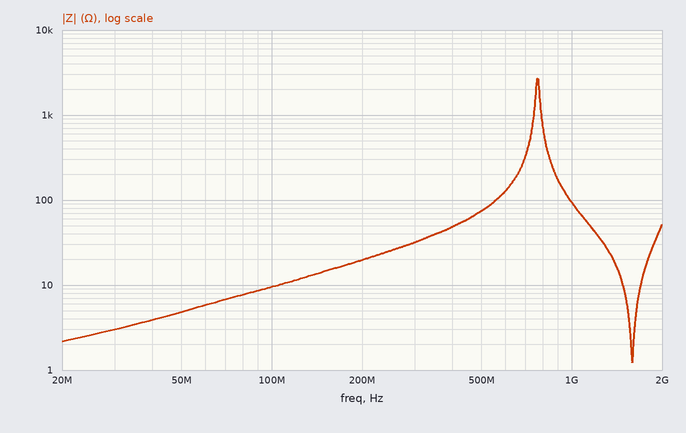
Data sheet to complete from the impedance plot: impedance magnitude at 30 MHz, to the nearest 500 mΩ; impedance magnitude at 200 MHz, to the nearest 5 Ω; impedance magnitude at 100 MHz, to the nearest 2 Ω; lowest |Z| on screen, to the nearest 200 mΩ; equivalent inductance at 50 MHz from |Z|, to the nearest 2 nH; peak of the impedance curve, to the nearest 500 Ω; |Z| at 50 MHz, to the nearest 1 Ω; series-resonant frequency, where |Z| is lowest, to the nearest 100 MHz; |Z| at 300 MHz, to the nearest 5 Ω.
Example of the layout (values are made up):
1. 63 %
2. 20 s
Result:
1. 3.0 Ω
2. 20 Ω
3. 10 Ω
4. 1.2 Ω
5. 16 nH
6. 2.5 kΩ
7. 5 Ω
8. 1.6 GHz
9. 30 Ω
